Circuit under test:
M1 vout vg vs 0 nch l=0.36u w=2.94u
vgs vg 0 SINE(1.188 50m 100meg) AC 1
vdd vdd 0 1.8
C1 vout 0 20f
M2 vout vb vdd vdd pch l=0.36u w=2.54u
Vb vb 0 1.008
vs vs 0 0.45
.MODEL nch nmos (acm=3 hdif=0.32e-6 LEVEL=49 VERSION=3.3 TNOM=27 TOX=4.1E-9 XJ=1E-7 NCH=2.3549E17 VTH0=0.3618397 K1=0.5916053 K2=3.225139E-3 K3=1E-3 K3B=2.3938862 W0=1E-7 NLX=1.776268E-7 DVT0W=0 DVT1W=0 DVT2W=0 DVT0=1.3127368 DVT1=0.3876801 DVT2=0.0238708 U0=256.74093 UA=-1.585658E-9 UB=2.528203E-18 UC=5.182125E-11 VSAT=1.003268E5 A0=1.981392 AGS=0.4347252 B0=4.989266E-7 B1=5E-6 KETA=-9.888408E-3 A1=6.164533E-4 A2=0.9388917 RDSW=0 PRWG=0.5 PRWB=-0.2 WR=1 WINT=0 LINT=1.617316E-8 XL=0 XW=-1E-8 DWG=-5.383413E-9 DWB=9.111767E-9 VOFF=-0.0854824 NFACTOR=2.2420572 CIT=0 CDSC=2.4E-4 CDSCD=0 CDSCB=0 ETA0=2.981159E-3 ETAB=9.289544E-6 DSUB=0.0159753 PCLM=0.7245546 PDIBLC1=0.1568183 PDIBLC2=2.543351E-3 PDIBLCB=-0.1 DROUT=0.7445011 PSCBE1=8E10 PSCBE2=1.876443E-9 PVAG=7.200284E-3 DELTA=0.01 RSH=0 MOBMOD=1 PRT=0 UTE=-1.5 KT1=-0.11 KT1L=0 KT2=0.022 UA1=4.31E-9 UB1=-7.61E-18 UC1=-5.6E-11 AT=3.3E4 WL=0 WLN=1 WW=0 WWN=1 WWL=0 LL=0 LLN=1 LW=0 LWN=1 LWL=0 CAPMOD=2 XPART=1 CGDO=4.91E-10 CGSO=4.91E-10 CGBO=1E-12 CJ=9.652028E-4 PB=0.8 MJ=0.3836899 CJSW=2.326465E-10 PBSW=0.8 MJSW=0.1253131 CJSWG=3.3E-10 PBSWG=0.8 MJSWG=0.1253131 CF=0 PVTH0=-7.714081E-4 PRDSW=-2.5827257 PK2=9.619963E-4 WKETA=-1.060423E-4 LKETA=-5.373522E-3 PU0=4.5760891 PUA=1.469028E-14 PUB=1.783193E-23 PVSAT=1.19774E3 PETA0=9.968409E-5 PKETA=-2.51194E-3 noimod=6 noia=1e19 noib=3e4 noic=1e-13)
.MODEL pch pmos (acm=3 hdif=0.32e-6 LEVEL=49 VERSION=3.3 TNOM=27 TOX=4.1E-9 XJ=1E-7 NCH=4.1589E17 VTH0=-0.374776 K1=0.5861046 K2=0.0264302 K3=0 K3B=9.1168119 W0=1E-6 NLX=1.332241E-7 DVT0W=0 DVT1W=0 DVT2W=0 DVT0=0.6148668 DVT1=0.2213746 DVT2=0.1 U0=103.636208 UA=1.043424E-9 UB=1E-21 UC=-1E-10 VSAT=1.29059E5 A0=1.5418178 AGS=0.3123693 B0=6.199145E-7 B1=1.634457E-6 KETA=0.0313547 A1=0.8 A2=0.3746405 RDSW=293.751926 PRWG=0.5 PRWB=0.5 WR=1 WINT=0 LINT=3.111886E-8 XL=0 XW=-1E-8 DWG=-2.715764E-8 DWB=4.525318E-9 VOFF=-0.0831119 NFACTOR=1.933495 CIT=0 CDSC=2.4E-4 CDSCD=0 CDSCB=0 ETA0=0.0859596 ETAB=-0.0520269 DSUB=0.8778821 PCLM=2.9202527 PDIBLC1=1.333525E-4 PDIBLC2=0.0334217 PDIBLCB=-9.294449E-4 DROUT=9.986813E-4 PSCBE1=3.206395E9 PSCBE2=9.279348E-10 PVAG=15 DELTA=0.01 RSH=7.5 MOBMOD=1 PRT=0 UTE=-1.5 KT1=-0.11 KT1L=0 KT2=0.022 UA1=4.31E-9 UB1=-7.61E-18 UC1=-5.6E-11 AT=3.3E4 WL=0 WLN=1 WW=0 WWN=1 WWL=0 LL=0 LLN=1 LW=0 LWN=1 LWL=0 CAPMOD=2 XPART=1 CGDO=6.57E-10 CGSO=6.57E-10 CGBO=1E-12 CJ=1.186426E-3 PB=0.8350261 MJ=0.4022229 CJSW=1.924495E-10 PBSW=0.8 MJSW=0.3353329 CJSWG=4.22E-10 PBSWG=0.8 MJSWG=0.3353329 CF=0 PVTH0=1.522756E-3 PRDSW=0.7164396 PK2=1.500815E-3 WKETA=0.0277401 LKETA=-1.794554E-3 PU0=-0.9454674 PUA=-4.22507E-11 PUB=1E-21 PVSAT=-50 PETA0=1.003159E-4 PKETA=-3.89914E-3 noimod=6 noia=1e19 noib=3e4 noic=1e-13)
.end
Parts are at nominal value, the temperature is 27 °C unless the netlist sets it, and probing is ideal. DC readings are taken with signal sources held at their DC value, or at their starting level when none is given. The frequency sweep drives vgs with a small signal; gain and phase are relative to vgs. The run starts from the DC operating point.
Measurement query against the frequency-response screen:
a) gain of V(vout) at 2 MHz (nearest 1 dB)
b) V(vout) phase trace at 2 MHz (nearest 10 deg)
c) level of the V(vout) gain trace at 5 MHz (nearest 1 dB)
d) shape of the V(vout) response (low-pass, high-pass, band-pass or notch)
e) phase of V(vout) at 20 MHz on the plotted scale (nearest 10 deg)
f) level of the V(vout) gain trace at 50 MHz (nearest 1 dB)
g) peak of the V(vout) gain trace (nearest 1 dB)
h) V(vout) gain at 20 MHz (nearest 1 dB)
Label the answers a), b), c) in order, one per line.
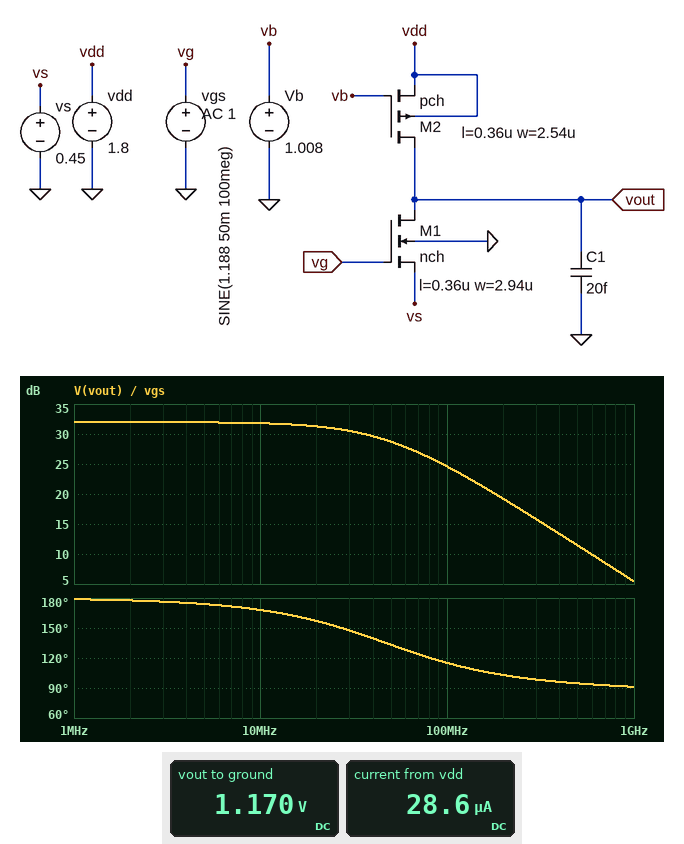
a) 32 dB
b) 180 deg
c) 32 dB
d) low-pass
e) 160 deg
f) 29 dB
g) 32 dB
h) 31 dB
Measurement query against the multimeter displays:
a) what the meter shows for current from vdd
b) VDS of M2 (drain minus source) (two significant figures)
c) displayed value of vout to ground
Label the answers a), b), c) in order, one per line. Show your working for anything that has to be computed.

a) 28.6 µA
b) 1.17 V - 1.8 V = -630 mV
c) 1.170 V
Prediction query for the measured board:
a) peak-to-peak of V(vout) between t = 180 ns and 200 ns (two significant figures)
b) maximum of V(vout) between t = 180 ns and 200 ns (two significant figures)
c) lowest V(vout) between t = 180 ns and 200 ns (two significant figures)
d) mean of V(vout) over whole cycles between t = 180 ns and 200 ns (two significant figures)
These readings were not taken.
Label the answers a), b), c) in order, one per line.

a) 1.1 V
b) 1.7 V
c) 540 mV
d) 1.1 V
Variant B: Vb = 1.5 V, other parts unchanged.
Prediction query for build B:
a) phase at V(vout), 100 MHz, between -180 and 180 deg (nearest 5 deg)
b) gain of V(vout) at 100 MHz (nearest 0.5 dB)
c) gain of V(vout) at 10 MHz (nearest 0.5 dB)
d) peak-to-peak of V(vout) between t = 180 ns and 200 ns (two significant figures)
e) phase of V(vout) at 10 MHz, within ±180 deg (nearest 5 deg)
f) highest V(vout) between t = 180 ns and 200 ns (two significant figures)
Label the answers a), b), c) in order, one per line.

a) 90 deg
b) -40.0 dB
c) -59.5 dB
d) 1.1 mV
e) 110 deg
f) 450 mV
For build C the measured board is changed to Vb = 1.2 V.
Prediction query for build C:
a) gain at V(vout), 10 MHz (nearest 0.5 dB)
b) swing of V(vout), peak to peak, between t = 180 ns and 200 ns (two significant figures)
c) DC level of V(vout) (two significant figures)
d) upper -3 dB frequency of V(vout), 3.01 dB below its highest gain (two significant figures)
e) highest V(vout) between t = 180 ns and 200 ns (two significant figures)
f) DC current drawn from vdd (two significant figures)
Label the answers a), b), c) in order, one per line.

a) -14.0 dB
b) 25 mV
c) 470 mV
d) 4.4 GHz
e) 490 mV
f) 6.9 µA
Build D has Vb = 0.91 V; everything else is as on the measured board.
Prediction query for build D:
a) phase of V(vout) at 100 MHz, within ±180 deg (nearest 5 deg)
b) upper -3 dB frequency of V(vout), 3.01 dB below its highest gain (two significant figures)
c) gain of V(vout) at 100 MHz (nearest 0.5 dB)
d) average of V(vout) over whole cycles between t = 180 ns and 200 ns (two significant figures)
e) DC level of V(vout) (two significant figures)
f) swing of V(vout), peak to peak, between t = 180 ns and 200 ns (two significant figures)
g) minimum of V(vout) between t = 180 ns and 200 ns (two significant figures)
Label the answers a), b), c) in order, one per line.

a) 170 deg
b) 580 MHz
c) 9.5 dB
d) 1.5 V
e) 1.6 V
f) 530 mV
g) 1.2 V
